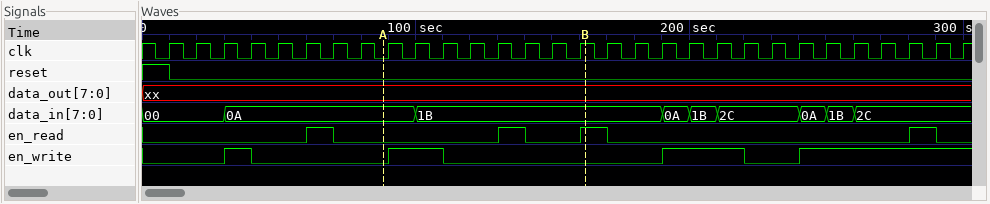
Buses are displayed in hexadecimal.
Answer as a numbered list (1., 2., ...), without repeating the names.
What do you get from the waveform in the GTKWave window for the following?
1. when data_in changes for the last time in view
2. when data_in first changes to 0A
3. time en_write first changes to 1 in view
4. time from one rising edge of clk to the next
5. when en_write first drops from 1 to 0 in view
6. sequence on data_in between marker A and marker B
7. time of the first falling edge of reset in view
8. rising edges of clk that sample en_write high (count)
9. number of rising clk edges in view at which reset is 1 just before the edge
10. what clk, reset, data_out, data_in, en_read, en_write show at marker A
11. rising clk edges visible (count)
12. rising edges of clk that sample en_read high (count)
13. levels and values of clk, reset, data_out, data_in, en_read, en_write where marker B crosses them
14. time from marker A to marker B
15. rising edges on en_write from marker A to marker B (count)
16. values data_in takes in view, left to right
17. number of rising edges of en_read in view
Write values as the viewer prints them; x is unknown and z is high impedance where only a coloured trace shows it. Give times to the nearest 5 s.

1. 260 s
2. 30 s
3. 30 s
4. 10 s
5. 40 s
6. 0A, 1B
7. 10 s
8. 12
9. 1
10. clk=0, reset=0, data_out=xx, data_in=0A, en_read=0, en_write=0
11. 30
12. 4
13. clk=1, reset=0, data_out=xx, data_in=1B, en_read=1, en_write=0
14. 75 s
15. 1
16. 00, 0A, 1B, 0A, 1B, 2C, 0A, 1B, 2C
17. 4
